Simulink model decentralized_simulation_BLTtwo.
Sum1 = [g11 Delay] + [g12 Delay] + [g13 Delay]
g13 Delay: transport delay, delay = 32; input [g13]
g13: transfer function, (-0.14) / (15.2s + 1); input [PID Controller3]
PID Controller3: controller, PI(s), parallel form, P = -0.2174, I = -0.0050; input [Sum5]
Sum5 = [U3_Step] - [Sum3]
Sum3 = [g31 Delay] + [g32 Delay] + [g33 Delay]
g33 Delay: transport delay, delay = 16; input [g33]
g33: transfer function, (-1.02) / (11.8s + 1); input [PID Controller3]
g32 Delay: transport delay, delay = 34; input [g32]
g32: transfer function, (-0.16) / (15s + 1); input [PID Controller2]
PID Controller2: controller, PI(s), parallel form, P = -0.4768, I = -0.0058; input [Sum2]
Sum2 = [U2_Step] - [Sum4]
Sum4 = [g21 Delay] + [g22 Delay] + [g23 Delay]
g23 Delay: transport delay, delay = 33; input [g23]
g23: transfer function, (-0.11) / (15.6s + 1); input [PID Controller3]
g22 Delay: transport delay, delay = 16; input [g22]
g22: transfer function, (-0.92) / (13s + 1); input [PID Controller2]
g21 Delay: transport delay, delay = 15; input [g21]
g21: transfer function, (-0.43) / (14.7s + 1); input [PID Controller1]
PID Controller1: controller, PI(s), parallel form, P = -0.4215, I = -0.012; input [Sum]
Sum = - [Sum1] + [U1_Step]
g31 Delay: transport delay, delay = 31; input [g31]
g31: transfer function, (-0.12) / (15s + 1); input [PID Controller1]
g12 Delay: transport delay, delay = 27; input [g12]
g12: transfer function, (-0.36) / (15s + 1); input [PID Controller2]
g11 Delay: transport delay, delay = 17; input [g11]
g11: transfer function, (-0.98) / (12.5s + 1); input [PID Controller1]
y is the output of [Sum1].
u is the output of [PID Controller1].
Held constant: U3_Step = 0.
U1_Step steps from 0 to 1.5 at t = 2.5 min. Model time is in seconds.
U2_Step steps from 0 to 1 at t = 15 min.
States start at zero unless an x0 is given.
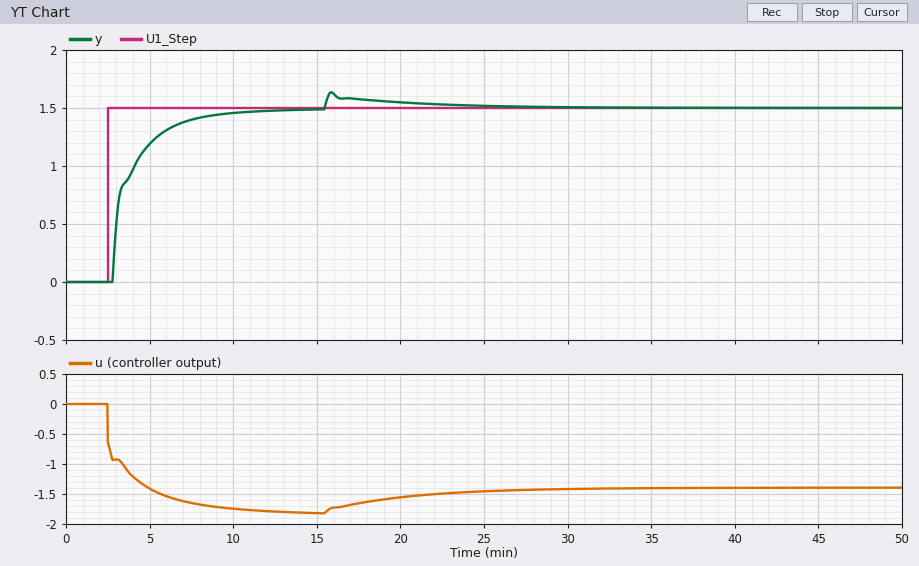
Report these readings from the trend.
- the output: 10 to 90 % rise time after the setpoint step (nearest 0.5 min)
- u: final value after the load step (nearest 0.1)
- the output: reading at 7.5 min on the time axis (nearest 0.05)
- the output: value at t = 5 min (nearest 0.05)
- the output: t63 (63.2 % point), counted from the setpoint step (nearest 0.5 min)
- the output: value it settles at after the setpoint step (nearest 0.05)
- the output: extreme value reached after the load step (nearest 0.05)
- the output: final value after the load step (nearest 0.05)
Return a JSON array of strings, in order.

["3.5 min", "-1.4", "1.40", "1.20", "1.5 min", "1.50", "1.65", "1.50"]
